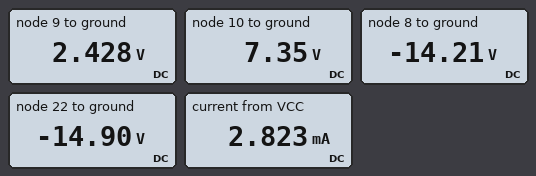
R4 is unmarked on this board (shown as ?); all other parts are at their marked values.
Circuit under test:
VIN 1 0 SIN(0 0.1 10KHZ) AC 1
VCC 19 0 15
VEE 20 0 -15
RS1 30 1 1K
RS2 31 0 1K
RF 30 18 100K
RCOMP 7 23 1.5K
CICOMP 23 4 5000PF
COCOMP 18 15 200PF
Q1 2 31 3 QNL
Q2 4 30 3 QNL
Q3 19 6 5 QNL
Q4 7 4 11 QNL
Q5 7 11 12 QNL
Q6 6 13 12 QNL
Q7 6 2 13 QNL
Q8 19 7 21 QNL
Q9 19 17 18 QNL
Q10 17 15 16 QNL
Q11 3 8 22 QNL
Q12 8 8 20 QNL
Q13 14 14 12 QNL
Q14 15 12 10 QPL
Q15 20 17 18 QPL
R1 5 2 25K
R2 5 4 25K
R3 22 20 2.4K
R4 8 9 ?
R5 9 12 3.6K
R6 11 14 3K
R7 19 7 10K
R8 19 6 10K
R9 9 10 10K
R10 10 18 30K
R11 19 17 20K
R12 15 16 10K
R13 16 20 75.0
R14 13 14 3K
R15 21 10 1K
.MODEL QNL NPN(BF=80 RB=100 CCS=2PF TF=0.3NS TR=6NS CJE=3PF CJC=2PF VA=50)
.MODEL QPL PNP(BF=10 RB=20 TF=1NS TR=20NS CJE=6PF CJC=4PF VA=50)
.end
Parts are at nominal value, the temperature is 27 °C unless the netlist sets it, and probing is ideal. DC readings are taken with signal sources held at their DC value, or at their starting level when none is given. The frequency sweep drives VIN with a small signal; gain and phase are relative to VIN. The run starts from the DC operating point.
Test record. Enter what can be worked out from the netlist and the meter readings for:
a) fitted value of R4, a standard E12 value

10 kΩ
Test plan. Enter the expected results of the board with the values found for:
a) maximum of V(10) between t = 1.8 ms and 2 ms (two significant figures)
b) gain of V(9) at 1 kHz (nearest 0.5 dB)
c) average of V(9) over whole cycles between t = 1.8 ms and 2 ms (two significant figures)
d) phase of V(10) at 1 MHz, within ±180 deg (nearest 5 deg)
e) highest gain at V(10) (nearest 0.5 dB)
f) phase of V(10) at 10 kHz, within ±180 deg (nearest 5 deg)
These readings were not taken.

7.4 V
1.0 dB
2.4 V
5 deg
5.5 dB
80 deg
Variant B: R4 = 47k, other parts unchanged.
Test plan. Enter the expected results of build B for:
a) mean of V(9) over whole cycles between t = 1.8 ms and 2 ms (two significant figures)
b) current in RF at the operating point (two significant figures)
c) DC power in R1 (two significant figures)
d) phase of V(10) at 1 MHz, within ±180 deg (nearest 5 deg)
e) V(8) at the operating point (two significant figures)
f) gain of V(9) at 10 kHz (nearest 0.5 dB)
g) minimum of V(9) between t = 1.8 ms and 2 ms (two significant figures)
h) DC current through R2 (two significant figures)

9.9 V
560 nA
6.6 µW
0 deg
-14 V
1.0 dB
9.8 V
16 µA
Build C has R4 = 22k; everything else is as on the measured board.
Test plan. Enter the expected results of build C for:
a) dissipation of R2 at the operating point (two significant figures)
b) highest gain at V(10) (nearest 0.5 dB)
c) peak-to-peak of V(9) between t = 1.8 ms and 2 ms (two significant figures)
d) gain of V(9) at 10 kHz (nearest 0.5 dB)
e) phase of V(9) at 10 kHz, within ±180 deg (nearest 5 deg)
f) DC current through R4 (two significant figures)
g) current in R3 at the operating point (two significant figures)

8.8 µW
5.0 dB
150 mV
0.5 dB
80 deg
960 µA
38 µA
